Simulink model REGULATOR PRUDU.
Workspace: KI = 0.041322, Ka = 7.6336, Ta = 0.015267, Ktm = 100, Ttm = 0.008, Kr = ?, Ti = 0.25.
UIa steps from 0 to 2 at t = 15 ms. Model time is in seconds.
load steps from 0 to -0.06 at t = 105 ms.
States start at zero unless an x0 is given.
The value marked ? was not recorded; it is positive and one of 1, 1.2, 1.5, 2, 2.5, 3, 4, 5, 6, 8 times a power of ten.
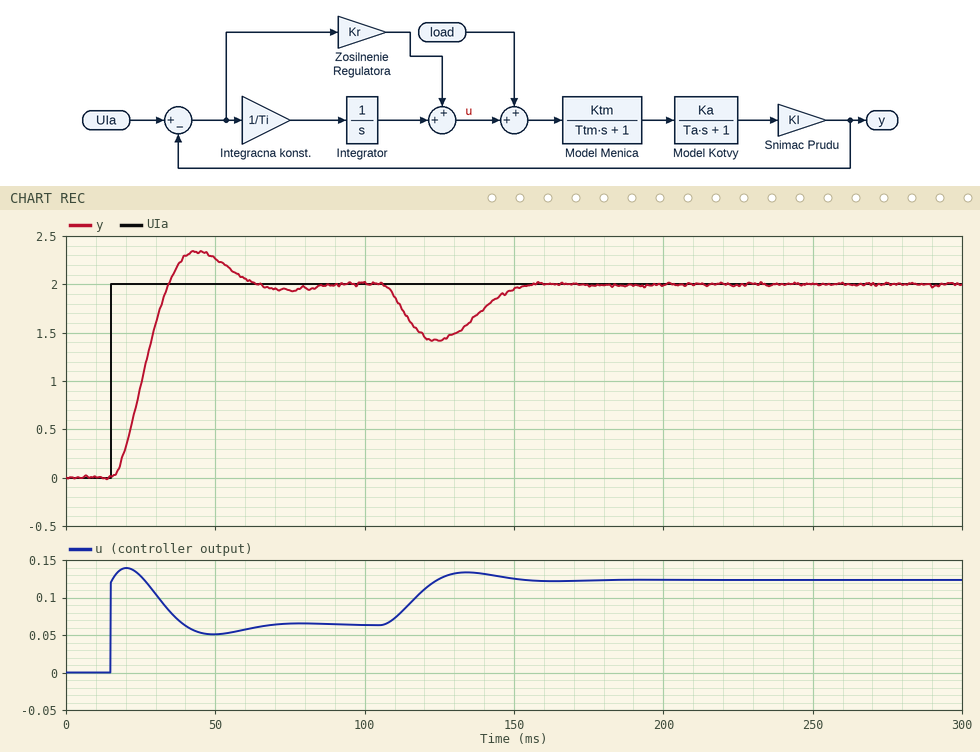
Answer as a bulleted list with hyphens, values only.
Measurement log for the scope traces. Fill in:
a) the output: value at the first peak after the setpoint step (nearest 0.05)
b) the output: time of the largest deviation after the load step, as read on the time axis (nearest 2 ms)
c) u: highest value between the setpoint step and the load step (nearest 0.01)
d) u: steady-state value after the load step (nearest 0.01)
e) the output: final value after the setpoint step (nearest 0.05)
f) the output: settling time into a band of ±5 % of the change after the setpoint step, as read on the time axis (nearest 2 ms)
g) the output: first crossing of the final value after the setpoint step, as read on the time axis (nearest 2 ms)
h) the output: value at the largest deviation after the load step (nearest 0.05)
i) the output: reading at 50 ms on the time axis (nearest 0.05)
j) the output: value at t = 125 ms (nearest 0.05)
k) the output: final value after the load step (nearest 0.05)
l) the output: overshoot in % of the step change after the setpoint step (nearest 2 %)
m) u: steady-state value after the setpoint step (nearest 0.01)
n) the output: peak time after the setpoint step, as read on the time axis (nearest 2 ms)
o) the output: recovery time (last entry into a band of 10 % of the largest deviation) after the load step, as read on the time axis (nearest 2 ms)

- 2.35
- 124 ms
- 0.14
- 0.12
- 2.00
- 58 ms
- 34 ms
- 1.40
- 2.25
- 1.40
- 2.00
- 16 %
- 0.06
- 44 ms
- 150 ms
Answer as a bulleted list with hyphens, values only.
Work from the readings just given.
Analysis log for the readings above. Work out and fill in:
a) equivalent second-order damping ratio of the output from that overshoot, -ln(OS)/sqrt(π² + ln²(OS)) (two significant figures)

- 0.50
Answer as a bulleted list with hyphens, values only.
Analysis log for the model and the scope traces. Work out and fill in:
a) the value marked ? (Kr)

- 0.06
